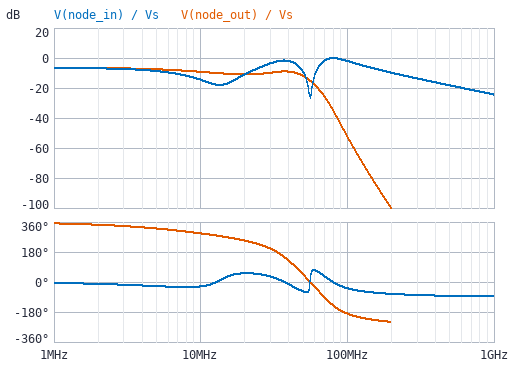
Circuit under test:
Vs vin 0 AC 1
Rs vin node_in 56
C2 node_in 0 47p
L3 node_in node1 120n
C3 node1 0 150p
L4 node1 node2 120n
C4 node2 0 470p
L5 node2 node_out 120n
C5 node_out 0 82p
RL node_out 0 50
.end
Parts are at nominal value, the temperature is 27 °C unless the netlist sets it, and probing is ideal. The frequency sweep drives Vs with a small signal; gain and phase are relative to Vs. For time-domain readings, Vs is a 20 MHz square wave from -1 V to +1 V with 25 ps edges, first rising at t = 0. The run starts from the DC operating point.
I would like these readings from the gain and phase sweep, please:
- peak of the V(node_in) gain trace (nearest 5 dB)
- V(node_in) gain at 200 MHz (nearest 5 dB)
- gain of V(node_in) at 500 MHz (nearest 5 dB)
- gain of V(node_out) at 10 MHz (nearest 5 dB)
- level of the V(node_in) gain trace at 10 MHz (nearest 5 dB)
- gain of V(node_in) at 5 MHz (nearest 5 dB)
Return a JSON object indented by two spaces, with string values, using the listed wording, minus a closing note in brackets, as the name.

{
  "peak of the V(node_in) gain trace": "0 dB",
  "V(node_in) gain at 200 MHz": "-10 dB",
  "gain of V(node_in) at 500 MHz": "-20 dB",
  "gain of V(node_out) at 10 MHz": "-10 dB",
  "level of the V(node_in) gain trace at 10 MHz": "-15 dB",
  "gain of V(node_in) at 5 MHz": "-10 dB"
}
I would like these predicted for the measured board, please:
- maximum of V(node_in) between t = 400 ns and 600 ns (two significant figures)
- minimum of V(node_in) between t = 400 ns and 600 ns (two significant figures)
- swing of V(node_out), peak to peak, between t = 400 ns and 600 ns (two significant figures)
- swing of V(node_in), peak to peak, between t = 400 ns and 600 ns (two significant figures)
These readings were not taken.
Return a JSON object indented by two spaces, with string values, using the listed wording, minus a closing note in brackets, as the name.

{
  "maximum of V(node_in) between t = 400 ns and 600 ns": "740 mV",
  "minimum of V(node_in) between t = 400 ns and 600 ns": "-740 mV",
  "swing of V(node_out), peak to peak, between t = 400 ns and 600 ns": "730 mV",
  "swing of V(node_in), peak to peak, between t = 400 ns and 600 ns": "1.5 V"
}
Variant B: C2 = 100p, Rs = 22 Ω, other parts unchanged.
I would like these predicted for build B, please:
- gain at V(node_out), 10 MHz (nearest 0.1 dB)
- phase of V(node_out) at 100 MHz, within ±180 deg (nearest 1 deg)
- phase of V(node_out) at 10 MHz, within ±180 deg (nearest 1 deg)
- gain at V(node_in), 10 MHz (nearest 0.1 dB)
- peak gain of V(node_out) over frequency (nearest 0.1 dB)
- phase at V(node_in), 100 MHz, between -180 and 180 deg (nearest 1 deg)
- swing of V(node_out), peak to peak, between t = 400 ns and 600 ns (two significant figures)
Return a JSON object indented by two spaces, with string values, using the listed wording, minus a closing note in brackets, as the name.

{
  "gain at V(node_out), 10 MHz": "-3.3 dB",
  "phase of V(node_out) at 100 MHz, within ±180 deg": "162 deg",
  "phase of V(node_out) at 10 MHz, within ±180 deg": "-64 deg",
  "gain at V(node_in), 10 MHz": "-8.5 dB",
  "peak gain of V(node_out) over frequency": "-3.2 dB",
  "phase at V(node_in), 100 MHz, between -180 and 180 deg": "-46 deg",
  "swing of V(node_out), peak to peak, between t = 400 ns and 600 ns": "1.4 V"
}
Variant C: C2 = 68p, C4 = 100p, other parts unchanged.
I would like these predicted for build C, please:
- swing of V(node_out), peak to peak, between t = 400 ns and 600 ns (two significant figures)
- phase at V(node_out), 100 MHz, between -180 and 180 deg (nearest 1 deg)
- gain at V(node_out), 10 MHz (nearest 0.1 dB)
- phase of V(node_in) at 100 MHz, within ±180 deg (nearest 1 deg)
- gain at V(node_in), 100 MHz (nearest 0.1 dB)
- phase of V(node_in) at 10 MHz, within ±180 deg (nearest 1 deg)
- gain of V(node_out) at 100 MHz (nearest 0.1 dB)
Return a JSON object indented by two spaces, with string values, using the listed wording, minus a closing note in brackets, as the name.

{
  "swing of V(node_out), peak to peak, between t = 400 ns and 600 ns": "1.1 V",
  "phase at V(node_out), 100 MHz, between -180 and 180 deg": "155 deg",
  "gain at V(node_out), 10 MHz": "-7.2 dB",
  "phase of V(node_in) at 100 MHz, within ±180 deg": "-56 deg",
  "gain at V(node_in), 100 MHz": "-5.1 dB",
  "phase of V(node_in) at 10 MHz, within ±180 deg": "-18 deg",
  "gain of V(node_out) at 100 MHz": "-36.6 dB"
}
